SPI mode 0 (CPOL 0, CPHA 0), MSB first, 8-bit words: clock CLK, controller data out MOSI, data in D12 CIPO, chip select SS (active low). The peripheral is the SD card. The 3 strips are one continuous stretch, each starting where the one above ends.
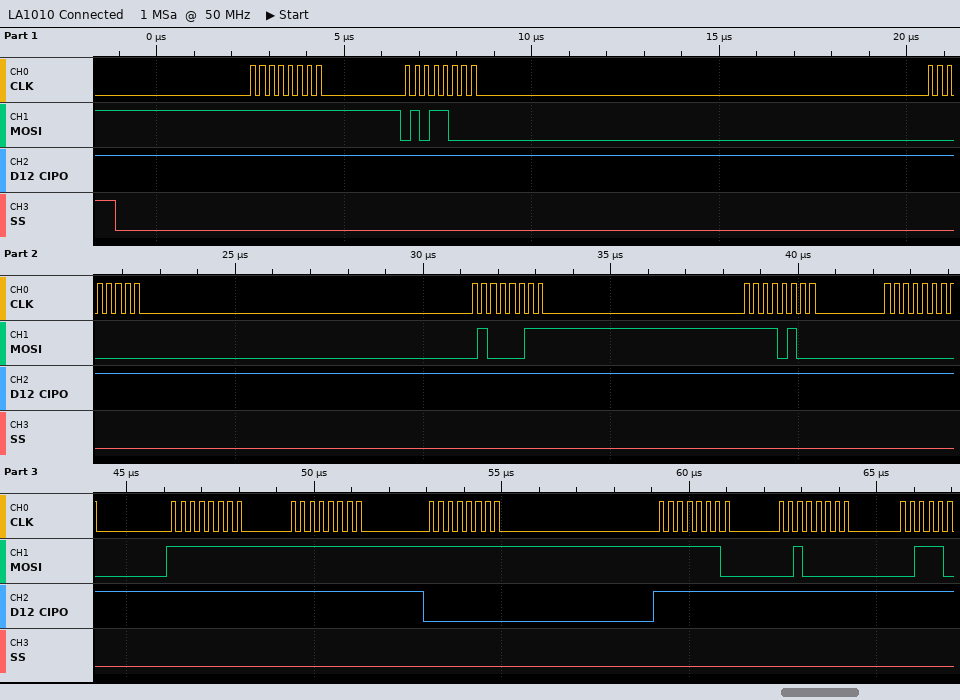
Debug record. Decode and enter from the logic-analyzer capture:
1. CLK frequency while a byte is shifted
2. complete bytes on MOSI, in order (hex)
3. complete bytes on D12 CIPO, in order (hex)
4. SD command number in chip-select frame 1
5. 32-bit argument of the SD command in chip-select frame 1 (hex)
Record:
4 MHz
FF 58 00 43 F4 00 FF FF FF FE 20
FF FF FF FF FF FF FF FF 00 FF FF
CMD24
0x0043F400
